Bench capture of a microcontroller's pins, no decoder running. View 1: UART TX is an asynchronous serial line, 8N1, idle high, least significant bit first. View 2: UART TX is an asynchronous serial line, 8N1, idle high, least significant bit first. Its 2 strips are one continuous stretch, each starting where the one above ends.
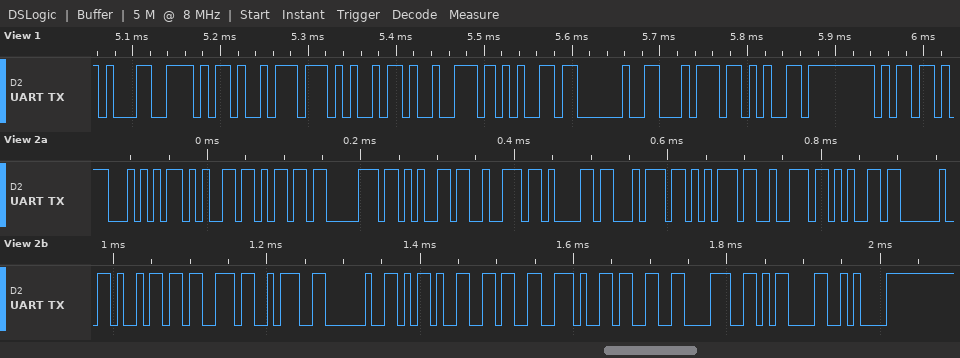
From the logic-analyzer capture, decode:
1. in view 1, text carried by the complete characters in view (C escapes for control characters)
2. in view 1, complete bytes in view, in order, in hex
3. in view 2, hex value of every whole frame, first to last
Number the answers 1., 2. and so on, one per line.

1. "1-wire tem"
2. 31 2D 77 69 72 65 20 74 65 6D
3. 54 65 6D 70 65 72 61 74 75 72 65 20 69 73 3A 20 2D 36 2E 33 38 0D 0A
